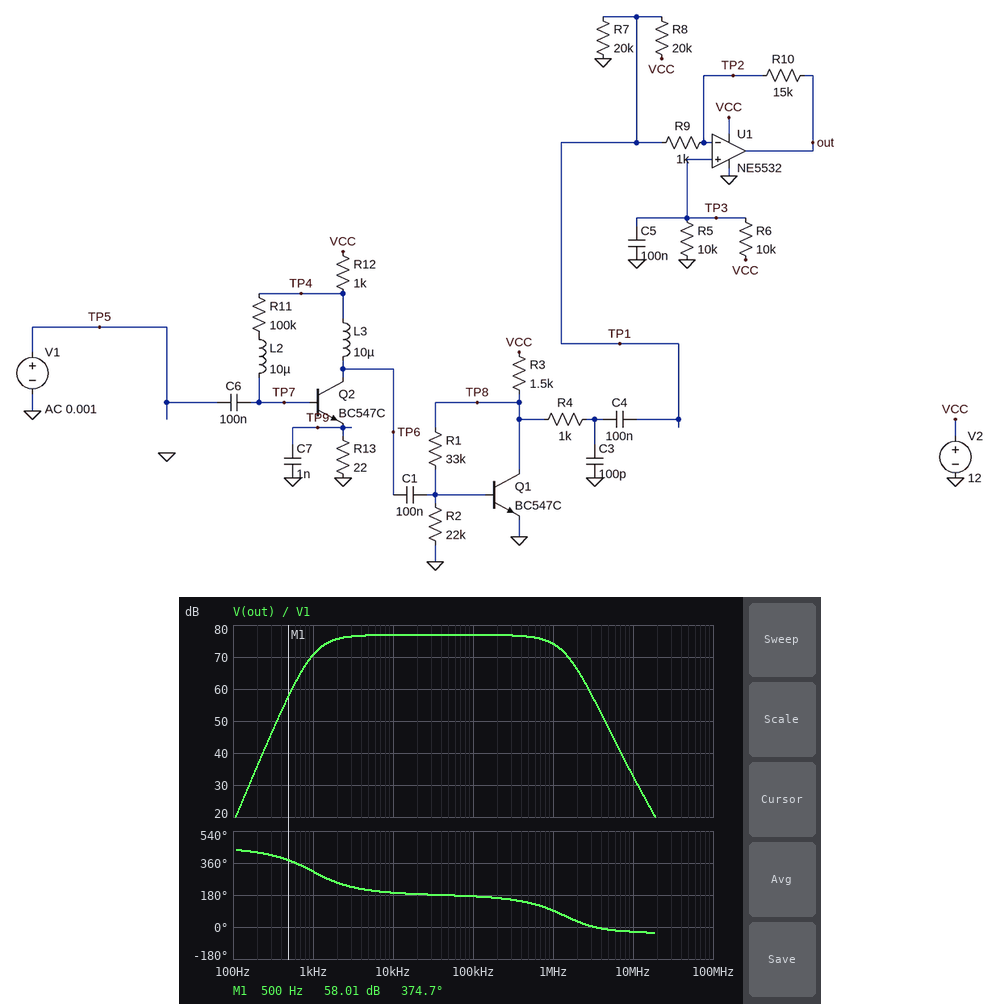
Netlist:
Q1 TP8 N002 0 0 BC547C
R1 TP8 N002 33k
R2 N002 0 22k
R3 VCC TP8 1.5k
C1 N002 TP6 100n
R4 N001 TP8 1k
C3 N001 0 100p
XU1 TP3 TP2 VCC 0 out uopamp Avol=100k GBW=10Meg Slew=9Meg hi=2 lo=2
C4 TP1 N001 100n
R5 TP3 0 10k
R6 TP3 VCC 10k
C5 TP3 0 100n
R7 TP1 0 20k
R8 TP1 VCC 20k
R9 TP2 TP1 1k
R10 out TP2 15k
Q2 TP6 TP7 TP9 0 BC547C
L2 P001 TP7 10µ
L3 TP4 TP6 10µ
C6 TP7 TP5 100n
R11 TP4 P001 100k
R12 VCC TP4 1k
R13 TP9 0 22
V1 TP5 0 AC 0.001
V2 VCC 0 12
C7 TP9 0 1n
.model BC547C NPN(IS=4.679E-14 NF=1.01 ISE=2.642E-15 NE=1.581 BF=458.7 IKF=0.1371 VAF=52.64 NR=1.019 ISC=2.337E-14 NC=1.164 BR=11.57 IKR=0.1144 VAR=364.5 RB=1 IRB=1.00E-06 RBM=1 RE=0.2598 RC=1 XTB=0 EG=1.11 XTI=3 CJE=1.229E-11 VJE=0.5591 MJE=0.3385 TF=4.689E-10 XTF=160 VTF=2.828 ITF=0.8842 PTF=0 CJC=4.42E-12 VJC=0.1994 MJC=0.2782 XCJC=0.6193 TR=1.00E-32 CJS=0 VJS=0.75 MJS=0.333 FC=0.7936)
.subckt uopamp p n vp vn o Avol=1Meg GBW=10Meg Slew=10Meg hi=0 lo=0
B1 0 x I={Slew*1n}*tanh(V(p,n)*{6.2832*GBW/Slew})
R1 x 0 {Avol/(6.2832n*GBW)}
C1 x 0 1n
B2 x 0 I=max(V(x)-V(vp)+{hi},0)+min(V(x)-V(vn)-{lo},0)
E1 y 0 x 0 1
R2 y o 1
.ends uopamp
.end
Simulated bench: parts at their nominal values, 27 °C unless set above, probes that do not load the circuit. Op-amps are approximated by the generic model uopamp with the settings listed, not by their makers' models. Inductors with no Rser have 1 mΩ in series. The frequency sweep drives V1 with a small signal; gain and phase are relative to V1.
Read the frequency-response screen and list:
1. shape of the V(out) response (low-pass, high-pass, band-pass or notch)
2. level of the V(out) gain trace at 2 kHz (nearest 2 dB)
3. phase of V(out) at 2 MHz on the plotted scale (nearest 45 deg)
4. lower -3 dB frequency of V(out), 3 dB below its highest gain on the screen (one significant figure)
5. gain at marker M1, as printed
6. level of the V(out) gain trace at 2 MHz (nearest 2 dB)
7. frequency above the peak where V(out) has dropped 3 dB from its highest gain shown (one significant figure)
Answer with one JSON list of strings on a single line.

["band-pass", "76 dB", "45 deg", "1 kHz", "58.01 dB", "66 dB", "1 MHz"]
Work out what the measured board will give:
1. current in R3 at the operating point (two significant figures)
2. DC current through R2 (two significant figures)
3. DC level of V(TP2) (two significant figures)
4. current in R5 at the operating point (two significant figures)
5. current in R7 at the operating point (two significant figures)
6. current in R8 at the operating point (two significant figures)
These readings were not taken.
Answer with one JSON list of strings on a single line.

["6.6 mA", "31 µA", "6.0 V", "600 µA", "300 µA", "300 µA"]
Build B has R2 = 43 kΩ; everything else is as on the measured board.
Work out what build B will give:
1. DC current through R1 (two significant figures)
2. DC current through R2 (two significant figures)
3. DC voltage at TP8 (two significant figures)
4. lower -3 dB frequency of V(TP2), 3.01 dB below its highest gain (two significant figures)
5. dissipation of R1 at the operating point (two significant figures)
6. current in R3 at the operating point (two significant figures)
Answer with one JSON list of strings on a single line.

["31 µA", "16 µA", "1.7 V", "570 kHz", "32 µW", "6.9 mA"]
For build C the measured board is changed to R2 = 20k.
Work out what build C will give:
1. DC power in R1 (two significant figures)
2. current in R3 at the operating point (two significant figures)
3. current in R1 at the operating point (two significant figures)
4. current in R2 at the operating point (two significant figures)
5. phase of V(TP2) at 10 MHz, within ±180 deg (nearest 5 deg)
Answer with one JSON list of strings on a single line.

["76 µW", "6.5 mA", "48 µA", "34 µA", "-115 deg"]
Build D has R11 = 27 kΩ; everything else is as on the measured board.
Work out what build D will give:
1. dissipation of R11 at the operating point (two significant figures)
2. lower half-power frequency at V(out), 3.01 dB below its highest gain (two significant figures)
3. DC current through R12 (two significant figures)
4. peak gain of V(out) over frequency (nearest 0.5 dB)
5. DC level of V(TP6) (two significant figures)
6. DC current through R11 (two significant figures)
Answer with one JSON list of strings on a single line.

["16 µW", "1.7 kHz", "10 mA", "77.5 dB", "1.6 V", "24 µA"]
